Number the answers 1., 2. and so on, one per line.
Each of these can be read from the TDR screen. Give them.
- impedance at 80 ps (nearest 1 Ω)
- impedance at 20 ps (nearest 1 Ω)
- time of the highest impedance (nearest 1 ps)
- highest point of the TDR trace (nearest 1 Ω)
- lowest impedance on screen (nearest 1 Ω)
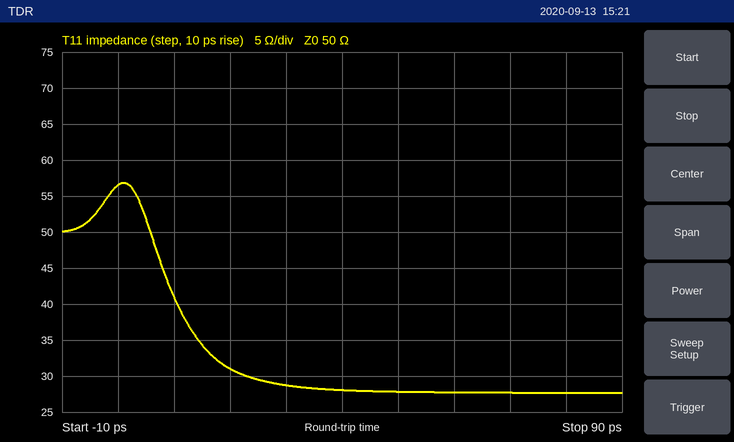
1. 28 Ω
2. 31 Ω
3. 1 ps
4. 57 Ω
5. 28 Ω
